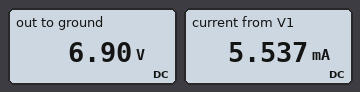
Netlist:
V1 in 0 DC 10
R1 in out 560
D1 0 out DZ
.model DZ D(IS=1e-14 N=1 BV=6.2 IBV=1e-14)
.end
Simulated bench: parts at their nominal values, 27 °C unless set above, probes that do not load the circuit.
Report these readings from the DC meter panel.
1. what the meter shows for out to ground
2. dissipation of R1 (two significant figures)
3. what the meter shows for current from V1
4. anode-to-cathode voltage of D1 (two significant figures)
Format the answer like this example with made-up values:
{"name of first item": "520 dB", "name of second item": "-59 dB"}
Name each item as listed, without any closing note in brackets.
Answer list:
{"what the meter shows for out to ground": "6.90 V", "dissipation of R1": "17 mW", "what the meter shows for current from V1": "5.537 mA", "anode-to-cathode voltage of D1": "-6.9 V"}
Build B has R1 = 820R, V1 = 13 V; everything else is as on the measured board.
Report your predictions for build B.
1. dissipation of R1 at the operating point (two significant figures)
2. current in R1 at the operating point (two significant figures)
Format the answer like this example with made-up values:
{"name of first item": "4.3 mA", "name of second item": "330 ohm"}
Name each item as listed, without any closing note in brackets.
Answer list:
{"dissipation of R1 at the operating point": "45 mW", "current in R1 at the operating point": "7.4 mA"}
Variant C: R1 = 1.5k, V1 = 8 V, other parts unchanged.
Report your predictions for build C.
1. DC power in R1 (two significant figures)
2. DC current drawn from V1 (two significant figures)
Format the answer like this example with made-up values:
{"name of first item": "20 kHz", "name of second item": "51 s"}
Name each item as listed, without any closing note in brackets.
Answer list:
{"DC power in R1": "880 µW", "DC current drawn from V1": "770 µA"}
